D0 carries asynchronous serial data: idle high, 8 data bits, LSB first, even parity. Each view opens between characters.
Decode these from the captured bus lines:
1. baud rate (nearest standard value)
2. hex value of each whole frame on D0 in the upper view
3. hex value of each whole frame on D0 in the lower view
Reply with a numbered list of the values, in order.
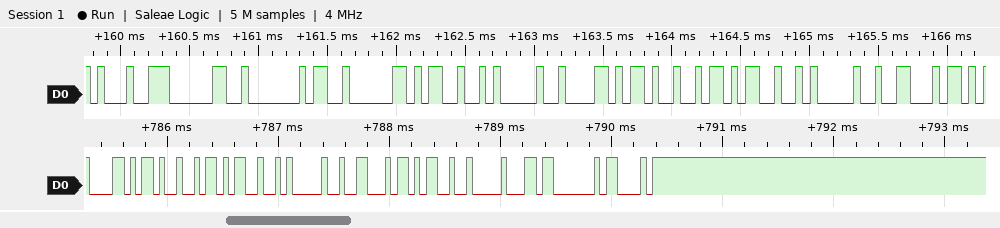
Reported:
1. 19200 baud
2. 91, 60, 40, 02, 4D, 41, 58, 49, 4D, 41, 46
3. 58, 49, 4D, 41, 46, 4D, 10, 03, 43
